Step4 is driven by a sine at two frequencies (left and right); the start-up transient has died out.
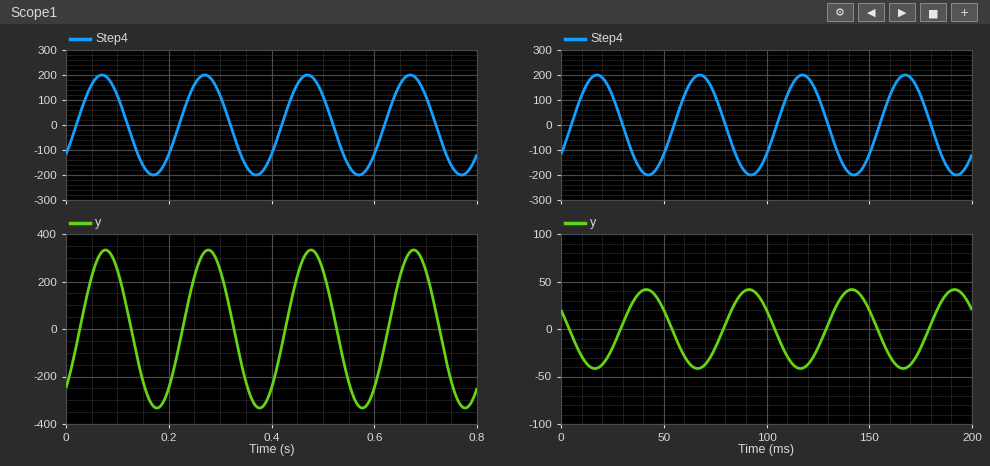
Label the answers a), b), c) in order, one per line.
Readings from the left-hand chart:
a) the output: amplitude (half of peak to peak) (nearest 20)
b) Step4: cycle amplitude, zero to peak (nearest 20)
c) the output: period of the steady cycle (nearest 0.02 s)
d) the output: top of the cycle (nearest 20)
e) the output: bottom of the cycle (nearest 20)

a) 340
b) 200
c) 0.20 s
d) 340
e) -340
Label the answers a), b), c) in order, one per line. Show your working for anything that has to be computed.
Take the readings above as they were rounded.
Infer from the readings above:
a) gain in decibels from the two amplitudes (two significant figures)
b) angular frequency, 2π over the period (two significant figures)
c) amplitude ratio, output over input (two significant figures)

a) 20 log10(340 / 200) = 4.6 dB
b) 2π / 0.2 = 31 rad/s
c) 340 / 200 = 1.7
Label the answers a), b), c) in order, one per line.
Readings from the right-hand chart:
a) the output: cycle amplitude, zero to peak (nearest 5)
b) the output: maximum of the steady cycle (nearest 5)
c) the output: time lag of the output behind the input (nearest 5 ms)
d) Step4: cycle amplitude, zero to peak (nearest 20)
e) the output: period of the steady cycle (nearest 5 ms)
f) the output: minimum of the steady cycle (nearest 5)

a) 40
b) 40
c) 25 ms
d) 200
e) 50 ms
f) -40
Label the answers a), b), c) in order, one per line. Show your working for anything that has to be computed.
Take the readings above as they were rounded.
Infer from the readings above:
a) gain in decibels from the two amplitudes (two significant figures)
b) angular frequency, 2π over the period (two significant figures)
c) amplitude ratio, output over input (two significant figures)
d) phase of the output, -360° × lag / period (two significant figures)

a) 20 log10(40 / 200) = -14 dB
b) 2π / 50 = 0.13 rad/ms
c) 40 / 200 = 0.20
d) -360 × 25 / 50 = -180°
